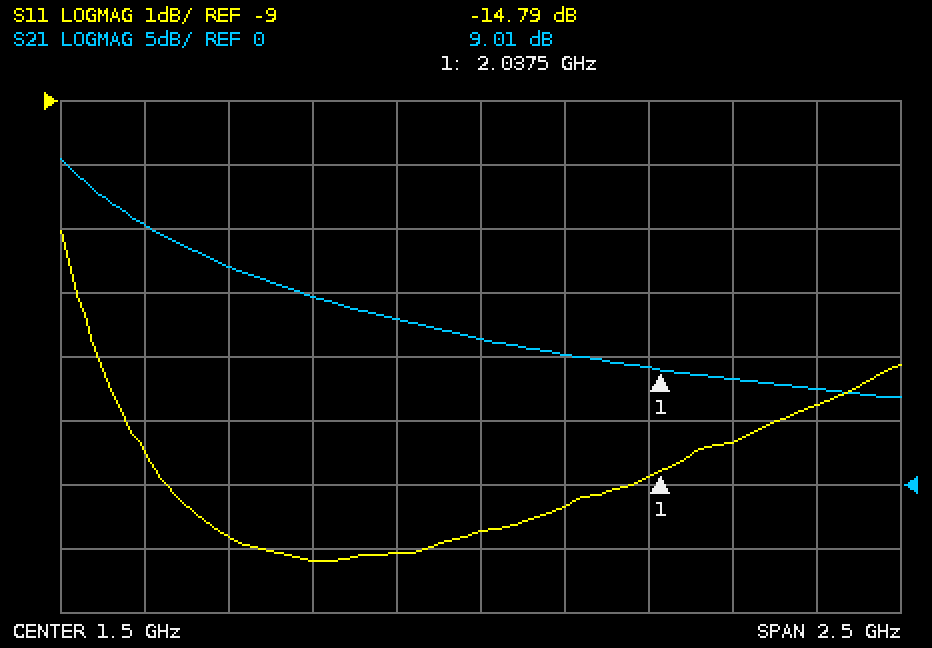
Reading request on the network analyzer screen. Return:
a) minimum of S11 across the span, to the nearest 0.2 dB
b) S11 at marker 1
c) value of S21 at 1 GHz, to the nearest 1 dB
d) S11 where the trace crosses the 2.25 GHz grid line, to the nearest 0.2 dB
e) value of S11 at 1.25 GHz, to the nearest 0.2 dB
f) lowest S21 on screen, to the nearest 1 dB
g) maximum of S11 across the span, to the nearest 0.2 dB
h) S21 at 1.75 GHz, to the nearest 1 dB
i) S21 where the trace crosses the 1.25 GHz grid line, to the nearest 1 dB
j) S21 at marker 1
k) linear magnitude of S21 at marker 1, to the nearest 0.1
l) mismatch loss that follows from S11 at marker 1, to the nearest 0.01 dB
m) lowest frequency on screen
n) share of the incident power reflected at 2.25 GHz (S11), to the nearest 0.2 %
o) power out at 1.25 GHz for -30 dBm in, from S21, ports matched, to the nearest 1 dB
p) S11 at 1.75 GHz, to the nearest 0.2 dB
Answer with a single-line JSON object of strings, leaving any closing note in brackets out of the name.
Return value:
{"minimum of S11 across the span, to the nearest 0.2 dB": "-16.2 dB", "S11 at marker 1": "-14.79 dB", "value of S21 at 1 GHz, to the nearest 1 dB": "15 dB", "S11 where the trace crosses the 2.25 GHz grid line, to the nearest 0.2 dB": "-14.4 dB", "value of S11 at 1.25 GHz, to the nearest 0.2 dB": "-16.0 dB", "lowest S21 on screen, to the nearest 1 dB": "7 dB", "maximum of S11 across the span, to the nearest 0.2 dB": "-11.0 dB", "S21 at 1.75 GHz, to the nearest 1 dB": "10 dB", "S21 where the trace crosses the 1.25 GHz grid line, to the nearest 1 dB": "13 dB", "S21 at marker 1": "9.01 dB", "linear magnitude of S21 at marker 1, to the nearest 0.1": "2.8", "mismatch loss that follows from S11 at marker 1, to the nearest 0.01 dB": "0.15 dB", "lowest frequency on screen": "250 MHz", "share of the incident power reflected at 2.25 GHz (S11), to the nearest 0.2 %": "3.6 %", "power out at 1.25 GHz for -30 dBm in, from S21, ports matched, to the nearest 1 dB": "-17 dBm", "S11 at 1.75 GHz, to the nearest 0.2 dB": "-15.4 dB"}
